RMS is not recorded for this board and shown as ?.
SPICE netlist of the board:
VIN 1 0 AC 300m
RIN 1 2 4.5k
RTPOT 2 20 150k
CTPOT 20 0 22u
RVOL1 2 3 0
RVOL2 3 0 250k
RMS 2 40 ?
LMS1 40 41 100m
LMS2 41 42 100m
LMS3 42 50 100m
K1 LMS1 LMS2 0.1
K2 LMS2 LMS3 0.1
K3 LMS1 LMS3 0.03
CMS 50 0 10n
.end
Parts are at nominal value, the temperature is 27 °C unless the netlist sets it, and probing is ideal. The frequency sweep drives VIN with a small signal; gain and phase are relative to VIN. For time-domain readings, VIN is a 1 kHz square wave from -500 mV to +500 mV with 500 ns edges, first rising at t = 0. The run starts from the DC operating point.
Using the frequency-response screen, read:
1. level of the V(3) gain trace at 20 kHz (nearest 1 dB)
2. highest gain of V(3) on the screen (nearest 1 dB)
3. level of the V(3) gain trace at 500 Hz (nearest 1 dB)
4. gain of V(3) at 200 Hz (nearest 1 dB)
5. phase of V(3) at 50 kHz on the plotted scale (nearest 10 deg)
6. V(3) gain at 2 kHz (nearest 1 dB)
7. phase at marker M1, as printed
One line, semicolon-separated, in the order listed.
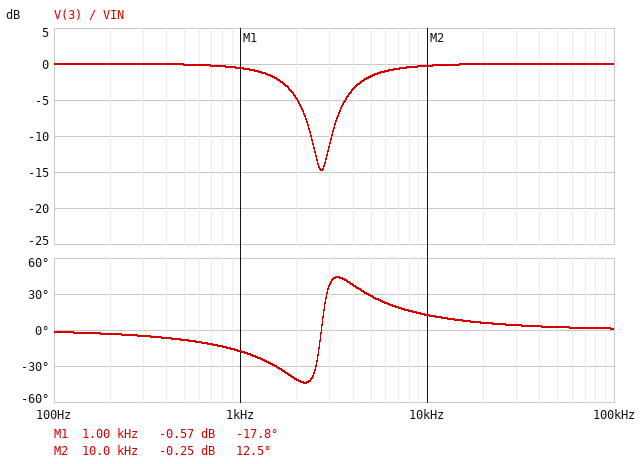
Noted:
0 dB; 0 dB; 0 dB; 0 dB; 0 deg; -5 dB; -17.8 deg
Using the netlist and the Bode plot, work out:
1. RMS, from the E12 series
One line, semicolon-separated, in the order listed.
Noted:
1 kΩ
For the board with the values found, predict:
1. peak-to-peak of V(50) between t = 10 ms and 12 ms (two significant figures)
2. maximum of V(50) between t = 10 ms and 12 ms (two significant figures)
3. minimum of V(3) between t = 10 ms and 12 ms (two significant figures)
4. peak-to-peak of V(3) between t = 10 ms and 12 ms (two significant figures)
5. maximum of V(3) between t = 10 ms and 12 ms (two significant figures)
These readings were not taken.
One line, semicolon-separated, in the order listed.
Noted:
1.4 V; 670 mV; -600 mV; 1.2 V; 570 mV
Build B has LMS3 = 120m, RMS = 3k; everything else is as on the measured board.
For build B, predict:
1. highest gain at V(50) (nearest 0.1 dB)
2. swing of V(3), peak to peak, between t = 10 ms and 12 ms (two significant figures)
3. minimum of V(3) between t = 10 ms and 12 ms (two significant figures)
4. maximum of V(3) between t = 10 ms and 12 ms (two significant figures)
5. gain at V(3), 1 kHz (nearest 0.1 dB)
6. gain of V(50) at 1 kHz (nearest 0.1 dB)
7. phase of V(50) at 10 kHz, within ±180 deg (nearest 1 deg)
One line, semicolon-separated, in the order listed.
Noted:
-1.1 dB; 870 mV; -440 mV; 420 mV; -2.6 dB; -1.5 dB; -163 deg
